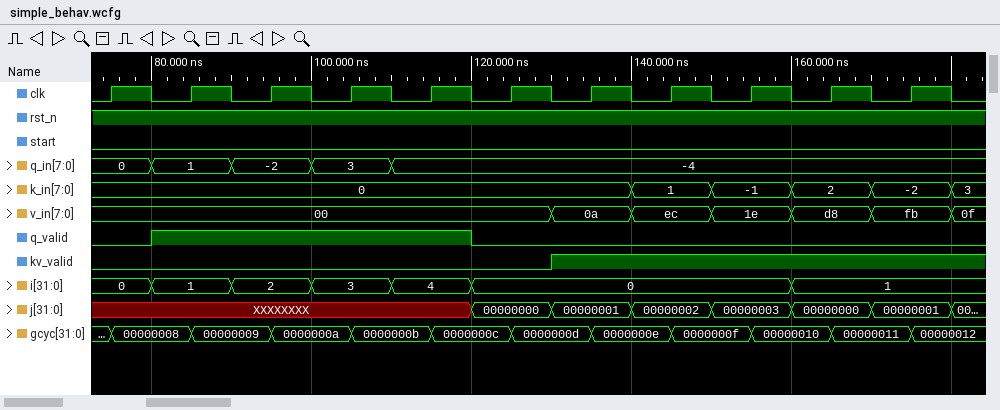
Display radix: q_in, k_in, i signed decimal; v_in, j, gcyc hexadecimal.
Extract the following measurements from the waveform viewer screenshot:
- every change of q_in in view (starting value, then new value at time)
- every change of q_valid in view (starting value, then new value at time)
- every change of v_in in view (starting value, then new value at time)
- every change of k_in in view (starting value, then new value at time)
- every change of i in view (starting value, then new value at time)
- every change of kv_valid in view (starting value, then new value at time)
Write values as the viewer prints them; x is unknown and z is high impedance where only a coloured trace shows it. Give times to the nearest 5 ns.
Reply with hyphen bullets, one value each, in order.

- 0, 1 at 80 ns, -2 at 90 ns, 3 at 100 ns, -4 at 110 ns
- 0, 1 at 80 ns, 0 at 120 ns
- 00, 0a at 130 ns, ec at 140 ns, 1e at 150 ns, d8 at 160 ns, fb at 170 ns, 0f at 180 ns
- 0, 1 at 140 ns, -1 at 150 ns, 2 at 160 ns, -2 at 170 ns, 3 at 180 ns
- 0, 1 at 80 ns, 2 at 90 ns, 3 at 100 ns, 4 at 110 ns, 0 at 120 ns, 1 at 160 ns
- 0, 1 at 130 ns
